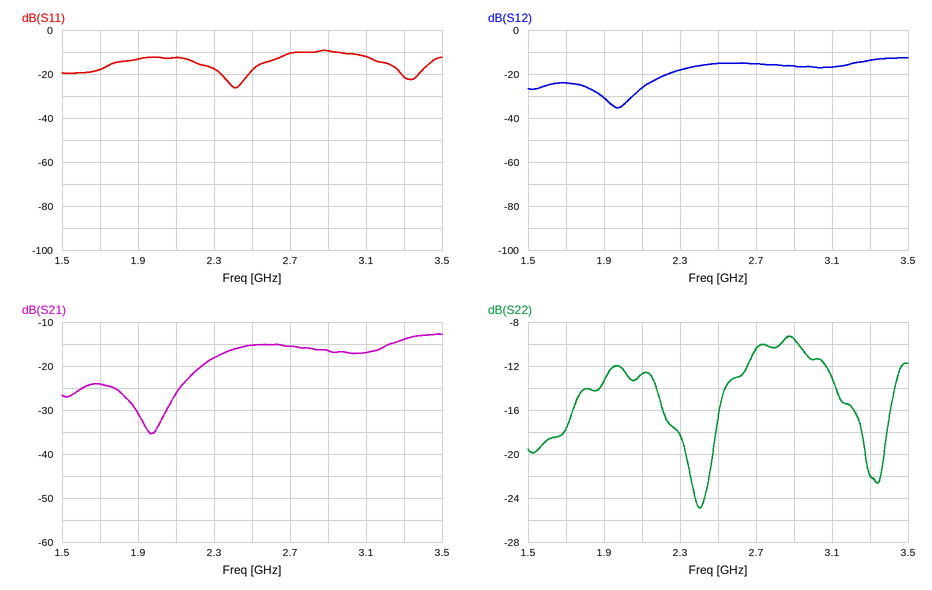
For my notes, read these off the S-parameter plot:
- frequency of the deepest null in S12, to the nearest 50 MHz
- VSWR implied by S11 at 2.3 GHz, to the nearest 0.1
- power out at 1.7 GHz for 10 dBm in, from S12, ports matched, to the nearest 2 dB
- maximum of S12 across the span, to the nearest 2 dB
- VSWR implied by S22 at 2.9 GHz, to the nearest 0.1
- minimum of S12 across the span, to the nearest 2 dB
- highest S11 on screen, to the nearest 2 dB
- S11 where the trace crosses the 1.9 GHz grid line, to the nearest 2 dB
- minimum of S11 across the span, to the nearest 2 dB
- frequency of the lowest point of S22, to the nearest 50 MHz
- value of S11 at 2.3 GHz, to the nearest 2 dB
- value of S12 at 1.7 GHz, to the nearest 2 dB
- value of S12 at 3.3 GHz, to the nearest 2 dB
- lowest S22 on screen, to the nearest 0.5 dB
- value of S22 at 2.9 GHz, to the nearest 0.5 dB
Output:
1.95 GHz
1.3
-14 dBm
-12 dB
2.0
-36 dB
-10 dB
-14 dB
-26 dB
2.40 GHz
-18 dB
-24 dB
-14 dB
-25.0 dB
-9.5 dB
